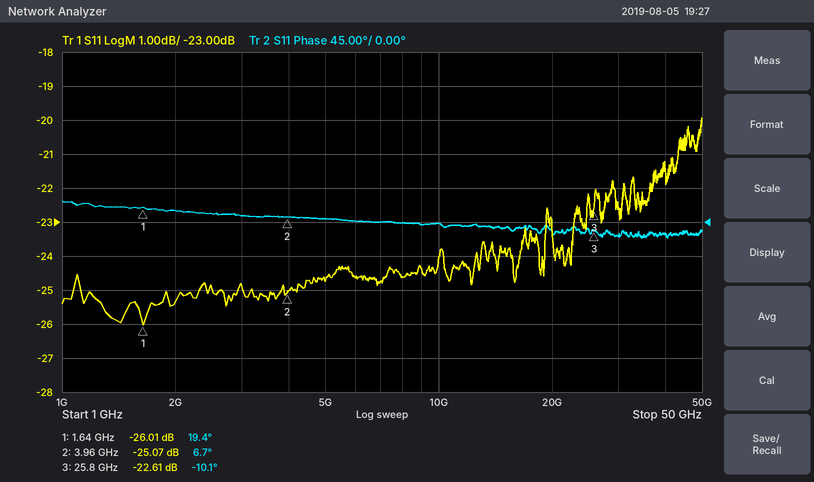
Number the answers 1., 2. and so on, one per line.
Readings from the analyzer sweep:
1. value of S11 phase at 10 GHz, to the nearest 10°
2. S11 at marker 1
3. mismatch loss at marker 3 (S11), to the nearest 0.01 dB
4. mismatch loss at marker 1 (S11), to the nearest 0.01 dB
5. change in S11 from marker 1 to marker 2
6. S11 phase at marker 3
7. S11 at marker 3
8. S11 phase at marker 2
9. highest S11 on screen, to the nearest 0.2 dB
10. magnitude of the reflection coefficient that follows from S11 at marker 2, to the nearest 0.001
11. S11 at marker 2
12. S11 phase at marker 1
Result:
1. 0°
2. -26.01 dB
3. 0.02 dB
4. 0.01 dB
5. 0.94 dB
6. -10.1°
7. -22.61 dB
8. 6.7°
9. -20.0 dB
10. 0.056
11. -25.07 dB
12. 19.4°
